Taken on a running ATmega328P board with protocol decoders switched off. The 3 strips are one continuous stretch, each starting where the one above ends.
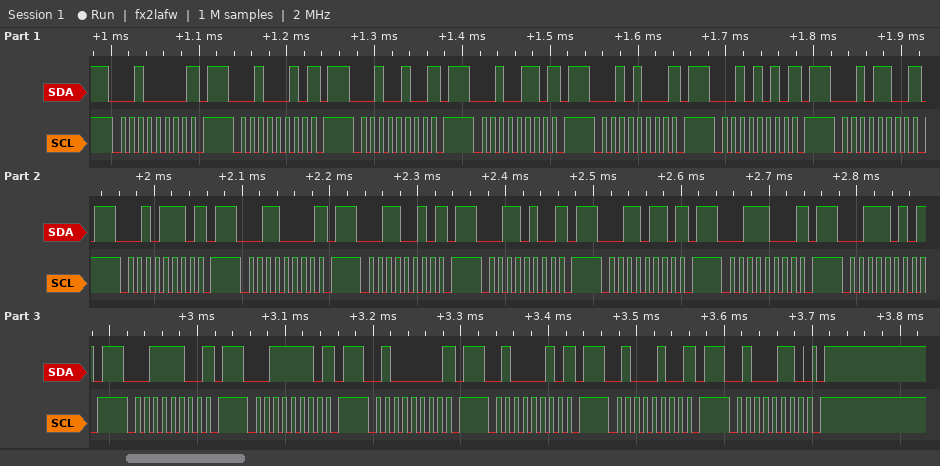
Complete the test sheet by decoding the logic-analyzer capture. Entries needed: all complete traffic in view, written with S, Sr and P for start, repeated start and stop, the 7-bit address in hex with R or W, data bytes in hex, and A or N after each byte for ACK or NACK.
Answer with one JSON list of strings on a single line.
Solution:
["S 10W N P S 11W N P S 12W N P S 13W N P S 14W N P S 15W N P S 16W N P S 17W N P S 18W N P S 19W N P S 1AW N P S 1BW N P S 1CW N P S 1DW N P S 1EW N P S 1FW N P S 20W N P S 21W N P S 22W N P S 23W A P"]
